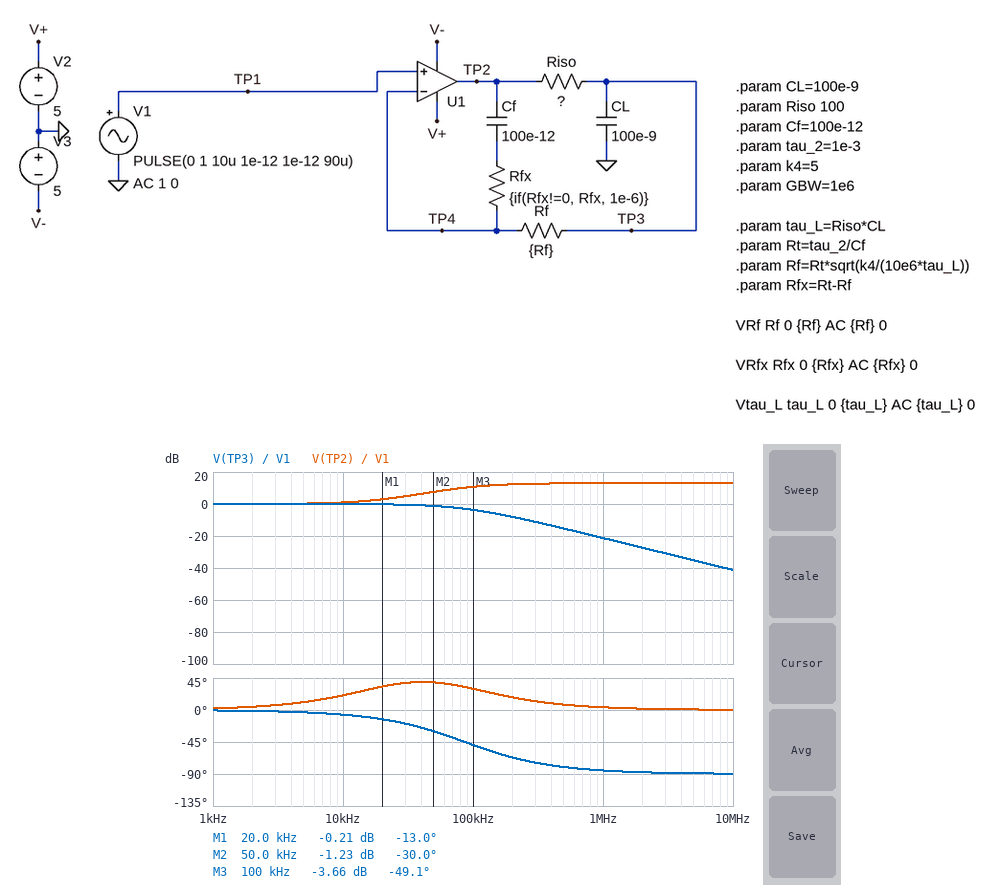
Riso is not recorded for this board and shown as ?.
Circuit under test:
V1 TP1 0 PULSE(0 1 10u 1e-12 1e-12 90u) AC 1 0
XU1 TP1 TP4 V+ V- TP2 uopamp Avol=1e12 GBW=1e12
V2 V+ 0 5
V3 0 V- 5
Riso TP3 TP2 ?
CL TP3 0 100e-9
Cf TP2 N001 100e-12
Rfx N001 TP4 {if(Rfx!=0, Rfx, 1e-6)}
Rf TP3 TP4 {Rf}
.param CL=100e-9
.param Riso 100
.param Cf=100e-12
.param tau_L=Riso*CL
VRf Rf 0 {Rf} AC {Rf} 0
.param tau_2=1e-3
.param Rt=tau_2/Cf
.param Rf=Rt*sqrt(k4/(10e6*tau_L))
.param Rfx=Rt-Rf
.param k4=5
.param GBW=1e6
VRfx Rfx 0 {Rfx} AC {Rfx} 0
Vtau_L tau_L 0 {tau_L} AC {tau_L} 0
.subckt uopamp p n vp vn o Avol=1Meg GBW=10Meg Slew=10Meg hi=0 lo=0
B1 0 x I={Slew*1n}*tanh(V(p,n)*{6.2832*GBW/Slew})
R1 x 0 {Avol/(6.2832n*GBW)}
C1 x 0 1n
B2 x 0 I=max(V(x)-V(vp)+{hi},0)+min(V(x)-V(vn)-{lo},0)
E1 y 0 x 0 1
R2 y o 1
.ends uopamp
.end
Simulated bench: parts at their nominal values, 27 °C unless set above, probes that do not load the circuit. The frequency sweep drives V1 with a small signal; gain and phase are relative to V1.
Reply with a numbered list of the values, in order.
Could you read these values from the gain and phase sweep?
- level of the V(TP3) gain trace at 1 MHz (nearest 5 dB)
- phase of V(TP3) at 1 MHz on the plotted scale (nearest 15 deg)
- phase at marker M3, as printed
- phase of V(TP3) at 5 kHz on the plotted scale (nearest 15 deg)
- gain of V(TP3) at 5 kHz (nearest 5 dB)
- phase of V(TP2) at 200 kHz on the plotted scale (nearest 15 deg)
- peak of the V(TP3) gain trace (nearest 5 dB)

1. -20 dB
2. -90 deg
3. -49.1 deg
4. 0 deg
5. 0 dB
6. 15 deg
7. 0 dB
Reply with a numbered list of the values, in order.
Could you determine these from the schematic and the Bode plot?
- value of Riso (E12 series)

1. 82 Ω
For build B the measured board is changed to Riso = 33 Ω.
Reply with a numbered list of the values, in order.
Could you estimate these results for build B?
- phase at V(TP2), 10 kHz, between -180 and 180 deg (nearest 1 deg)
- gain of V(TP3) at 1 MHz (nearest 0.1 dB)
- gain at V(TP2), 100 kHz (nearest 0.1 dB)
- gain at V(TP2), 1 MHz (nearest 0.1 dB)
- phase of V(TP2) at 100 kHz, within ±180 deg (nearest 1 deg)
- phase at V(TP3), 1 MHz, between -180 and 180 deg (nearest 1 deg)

1. 9 deg
2. -13.5 dB
3. 6.4 dB
4. 12.8 dB
5. 39 deg
6. -78 deg
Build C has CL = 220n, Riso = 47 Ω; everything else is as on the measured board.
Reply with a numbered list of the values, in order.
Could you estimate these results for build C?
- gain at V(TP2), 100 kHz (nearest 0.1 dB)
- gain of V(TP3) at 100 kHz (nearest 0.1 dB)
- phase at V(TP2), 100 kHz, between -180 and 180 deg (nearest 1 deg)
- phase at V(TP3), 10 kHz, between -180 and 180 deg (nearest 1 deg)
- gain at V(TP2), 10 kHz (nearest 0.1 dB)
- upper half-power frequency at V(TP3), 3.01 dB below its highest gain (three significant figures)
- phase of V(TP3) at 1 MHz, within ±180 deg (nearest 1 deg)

1. 11.4 dB
2. -4.9 dB
3. 26 deg
4. -8 deg
5. 1.5 dB
6. 68.7 kHz
7. -86 deg
